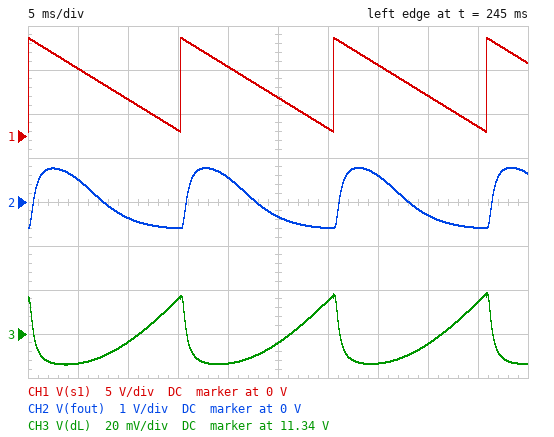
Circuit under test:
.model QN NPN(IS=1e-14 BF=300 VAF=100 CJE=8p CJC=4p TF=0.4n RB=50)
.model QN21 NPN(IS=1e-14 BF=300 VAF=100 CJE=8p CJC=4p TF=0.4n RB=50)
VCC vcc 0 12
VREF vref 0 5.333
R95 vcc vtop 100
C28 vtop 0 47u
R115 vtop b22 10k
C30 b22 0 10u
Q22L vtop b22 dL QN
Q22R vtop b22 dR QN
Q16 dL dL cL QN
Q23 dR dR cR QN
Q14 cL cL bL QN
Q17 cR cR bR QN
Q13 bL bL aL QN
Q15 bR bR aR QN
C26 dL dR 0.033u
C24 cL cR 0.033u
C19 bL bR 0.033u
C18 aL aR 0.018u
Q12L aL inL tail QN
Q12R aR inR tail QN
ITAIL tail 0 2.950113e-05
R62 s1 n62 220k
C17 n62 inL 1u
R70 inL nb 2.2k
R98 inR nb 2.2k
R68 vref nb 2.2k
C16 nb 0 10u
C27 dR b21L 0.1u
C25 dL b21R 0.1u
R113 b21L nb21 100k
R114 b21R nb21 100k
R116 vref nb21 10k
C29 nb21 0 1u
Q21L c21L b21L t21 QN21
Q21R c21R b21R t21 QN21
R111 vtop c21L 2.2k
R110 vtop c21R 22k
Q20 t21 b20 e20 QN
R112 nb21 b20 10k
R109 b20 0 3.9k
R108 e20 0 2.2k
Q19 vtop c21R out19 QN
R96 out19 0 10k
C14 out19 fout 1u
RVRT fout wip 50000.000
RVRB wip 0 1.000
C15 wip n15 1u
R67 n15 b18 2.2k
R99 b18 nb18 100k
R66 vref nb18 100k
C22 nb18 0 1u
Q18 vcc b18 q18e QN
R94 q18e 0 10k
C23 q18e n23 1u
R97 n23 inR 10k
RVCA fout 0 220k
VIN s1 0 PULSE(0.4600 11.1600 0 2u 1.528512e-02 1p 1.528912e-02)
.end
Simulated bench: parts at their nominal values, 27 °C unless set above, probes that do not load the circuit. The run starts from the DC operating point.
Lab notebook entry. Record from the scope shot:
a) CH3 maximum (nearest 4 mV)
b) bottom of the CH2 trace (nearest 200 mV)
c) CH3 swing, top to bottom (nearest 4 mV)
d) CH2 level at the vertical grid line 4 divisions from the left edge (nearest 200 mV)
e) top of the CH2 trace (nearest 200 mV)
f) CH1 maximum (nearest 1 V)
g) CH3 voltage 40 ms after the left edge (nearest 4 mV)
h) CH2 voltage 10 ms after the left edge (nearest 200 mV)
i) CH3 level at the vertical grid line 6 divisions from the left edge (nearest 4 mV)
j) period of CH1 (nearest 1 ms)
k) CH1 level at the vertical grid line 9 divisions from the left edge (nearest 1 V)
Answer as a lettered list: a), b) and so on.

a) 11.360 V
b) -600 mV
c) 32 mV
d) 600 mV
e) 800 mV
f) 11 V
g) 11.336 V
h) -400 mV
i) 11.356 V
j) 15 ms
k) 1 V
